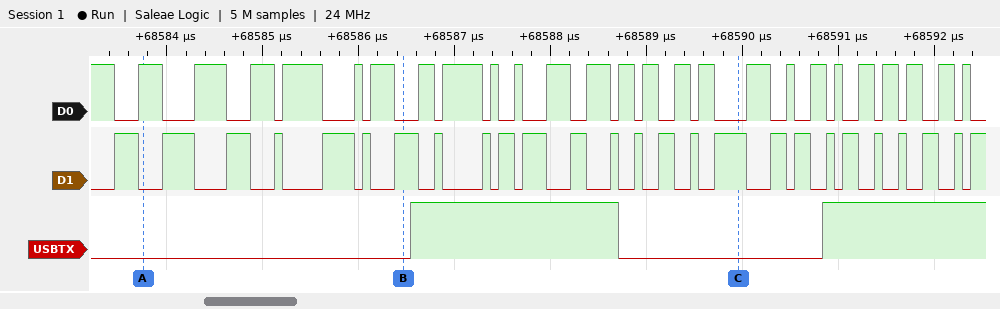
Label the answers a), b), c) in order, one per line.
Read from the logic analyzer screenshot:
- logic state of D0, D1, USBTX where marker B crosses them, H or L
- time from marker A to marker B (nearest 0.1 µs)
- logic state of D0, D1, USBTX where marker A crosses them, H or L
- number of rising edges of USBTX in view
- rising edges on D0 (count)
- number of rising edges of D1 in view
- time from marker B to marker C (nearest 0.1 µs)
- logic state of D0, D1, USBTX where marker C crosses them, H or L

a) D0=L, D1=H, USBTX=L
b) 2.7 µs
c) D0=H, D1=L, USBTX=L
d) 2
e) 25
f) 26
g) 3.5 µs
h) D0=L, D1=H, USBTX=L
